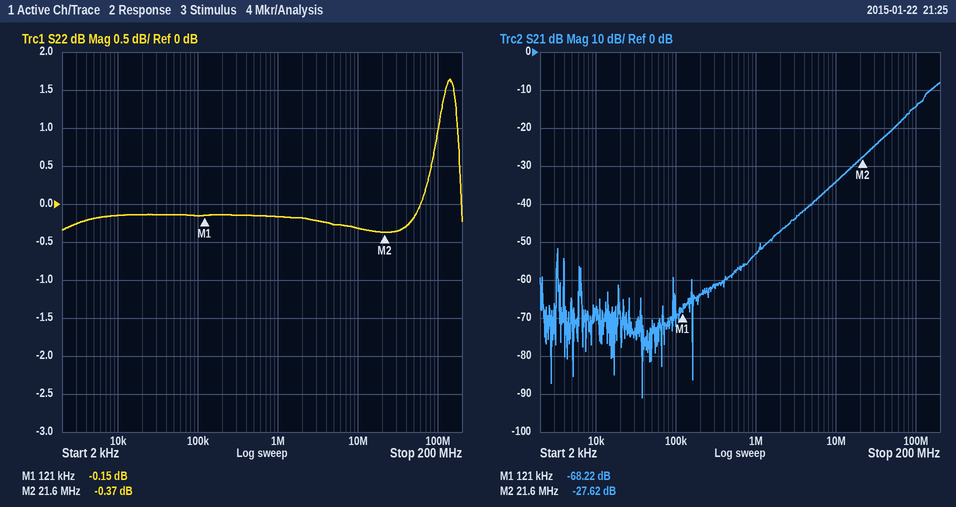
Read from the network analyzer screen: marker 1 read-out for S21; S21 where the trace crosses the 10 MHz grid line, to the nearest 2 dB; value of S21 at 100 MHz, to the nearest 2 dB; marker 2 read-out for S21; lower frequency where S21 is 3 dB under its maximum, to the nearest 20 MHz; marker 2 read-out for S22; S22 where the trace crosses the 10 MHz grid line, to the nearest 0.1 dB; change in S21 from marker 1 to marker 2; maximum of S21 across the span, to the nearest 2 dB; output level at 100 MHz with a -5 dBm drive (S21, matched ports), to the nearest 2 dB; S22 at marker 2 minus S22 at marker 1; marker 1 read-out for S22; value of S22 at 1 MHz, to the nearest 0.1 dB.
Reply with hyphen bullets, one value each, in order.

- -68.22 dB
- -34 dB
- -14 dB
- -27.62 dB
- 140 MHz
- -0.37 dB
- -0.3 dB
- 40.60 dB
- -8 dB
- -20 dBm
- -0.22 dB
- -0.15 dB
- -0.2 dB
